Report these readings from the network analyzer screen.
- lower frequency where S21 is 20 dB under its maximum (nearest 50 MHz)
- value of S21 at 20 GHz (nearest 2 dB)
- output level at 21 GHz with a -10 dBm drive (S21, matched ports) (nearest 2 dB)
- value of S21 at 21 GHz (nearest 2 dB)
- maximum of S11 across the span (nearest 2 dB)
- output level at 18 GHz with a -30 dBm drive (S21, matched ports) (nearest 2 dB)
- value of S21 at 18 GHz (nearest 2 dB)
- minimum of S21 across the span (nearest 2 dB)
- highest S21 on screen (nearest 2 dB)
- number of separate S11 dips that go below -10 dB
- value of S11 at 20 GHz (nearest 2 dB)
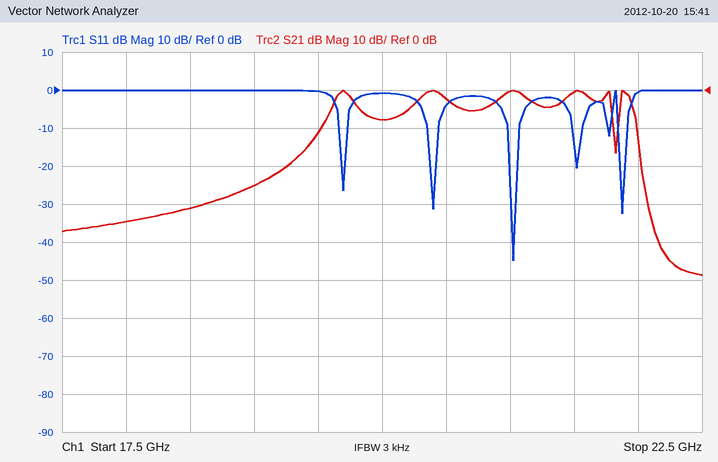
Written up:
19.25 GHz
-8 dB
-10 dBm
0 dB
0 dB
-64 dBm
-34 dB
-48 dB
0 dB
6
0 dB
